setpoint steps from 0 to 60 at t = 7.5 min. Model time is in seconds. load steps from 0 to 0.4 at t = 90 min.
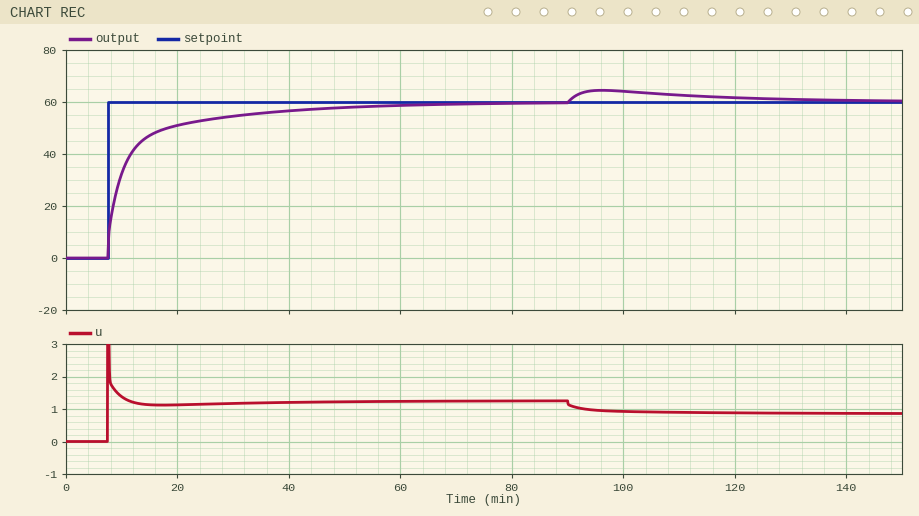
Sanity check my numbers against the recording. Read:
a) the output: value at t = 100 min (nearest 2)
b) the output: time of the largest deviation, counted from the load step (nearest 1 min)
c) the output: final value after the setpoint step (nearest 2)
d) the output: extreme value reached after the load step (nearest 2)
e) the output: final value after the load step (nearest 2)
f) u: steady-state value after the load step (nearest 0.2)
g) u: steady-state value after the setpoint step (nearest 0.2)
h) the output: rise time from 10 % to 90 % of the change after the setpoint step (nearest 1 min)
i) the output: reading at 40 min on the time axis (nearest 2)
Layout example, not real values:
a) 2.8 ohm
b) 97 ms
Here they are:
a) 64
b) 6 min
c) 60
d) 64
e) 60
f) 0.8
g) 1.2
h) 20 min
i) 56
